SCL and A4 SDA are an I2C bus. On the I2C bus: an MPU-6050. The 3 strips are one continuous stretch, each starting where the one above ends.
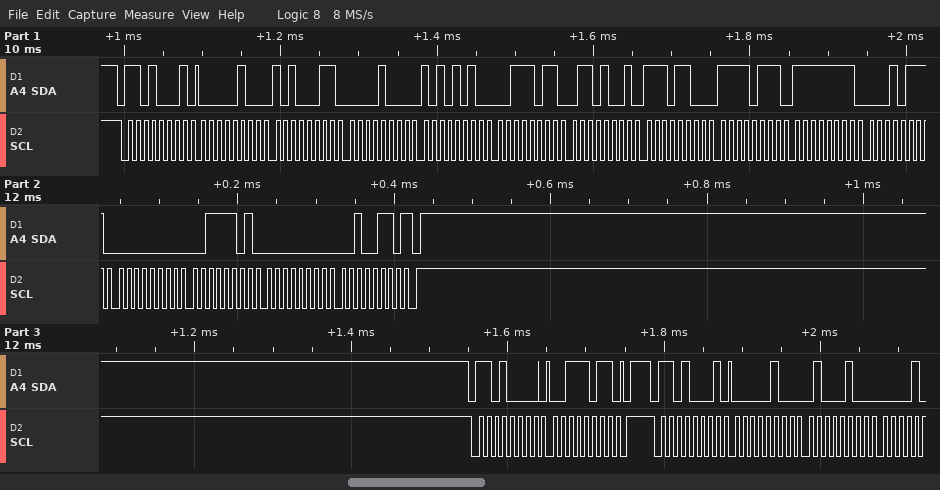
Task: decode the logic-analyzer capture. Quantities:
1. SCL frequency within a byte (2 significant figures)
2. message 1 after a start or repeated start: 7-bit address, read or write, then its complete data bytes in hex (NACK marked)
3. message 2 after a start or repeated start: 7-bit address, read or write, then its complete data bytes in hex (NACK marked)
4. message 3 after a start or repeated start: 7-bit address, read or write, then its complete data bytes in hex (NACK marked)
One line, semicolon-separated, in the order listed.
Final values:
100 kHz; 0x68 read: 04 A3 08 AA 3B 69 EC F7 FF 17 00 3D 00 26 NACK; 0x68 write: 3B; 0x68 read: 04 44
